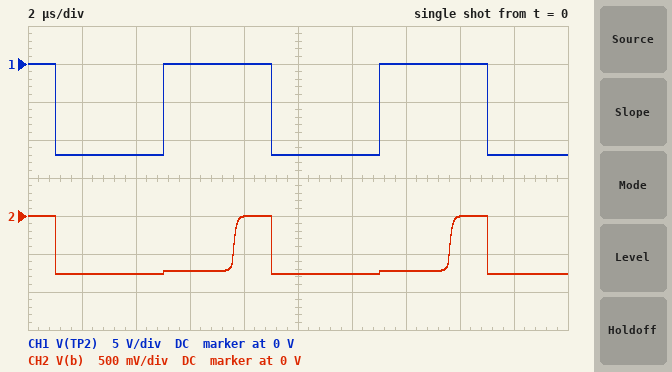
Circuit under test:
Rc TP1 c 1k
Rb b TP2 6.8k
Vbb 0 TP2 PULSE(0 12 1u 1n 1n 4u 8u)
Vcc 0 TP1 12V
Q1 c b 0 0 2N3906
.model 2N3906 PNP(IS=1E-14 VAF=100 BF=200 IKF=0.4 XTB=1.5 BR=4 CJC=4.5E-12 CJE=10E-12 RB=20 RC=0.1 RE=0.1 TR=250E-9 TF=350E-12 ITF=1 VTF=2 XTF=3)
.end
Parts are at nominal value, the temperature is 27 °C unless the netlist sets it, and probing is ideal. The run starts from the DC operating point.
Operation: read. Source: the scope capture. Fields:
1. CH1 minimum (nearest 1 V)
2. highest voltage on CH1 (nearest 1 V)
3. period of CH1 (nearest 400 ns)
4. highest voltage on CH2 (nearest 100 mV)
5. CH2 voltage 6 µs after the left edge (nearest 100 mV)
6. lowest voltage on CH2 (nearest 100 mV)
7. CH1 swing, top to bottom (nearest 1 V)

-12 V
0 V
8.0 µs
0 V
-700 mV
-800 mV
12 V
